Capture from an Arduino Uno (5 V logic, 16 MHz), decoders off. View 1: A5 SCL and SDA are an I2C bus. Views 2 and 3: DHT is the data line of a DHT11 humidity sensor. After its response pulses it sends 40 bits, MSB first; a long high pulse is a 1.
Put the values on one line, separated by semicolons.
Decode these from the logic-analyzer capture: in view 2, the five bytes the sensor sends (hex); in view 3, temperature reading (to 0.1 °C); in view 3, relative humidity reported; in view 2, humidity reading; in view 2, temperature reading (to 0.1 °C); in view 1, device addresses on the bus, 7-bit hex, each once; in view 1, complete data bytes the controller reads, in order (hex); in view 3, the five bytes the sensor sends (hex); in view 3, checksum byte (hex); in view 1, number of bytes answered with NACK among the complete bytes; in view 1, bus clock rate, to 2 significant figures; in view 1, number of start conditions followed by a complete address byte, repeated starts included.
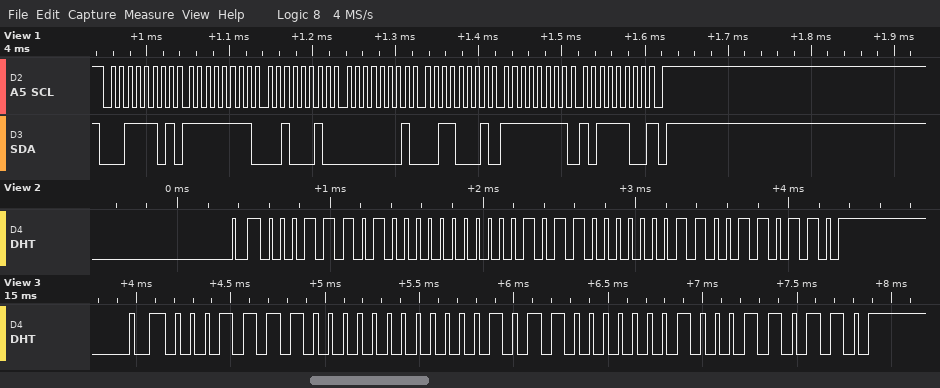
1D 00 16 03 36; 22.2 °C; 30 %; 29 %; 22.3 °C; 0x1E; FF 22 01 31 FF BC; 1E 00 16 02 36; 0x36; 1; 100 kHz; 1
